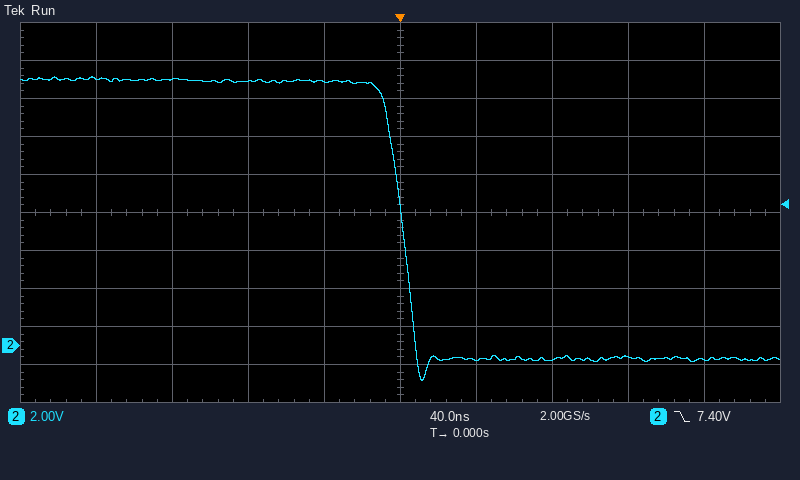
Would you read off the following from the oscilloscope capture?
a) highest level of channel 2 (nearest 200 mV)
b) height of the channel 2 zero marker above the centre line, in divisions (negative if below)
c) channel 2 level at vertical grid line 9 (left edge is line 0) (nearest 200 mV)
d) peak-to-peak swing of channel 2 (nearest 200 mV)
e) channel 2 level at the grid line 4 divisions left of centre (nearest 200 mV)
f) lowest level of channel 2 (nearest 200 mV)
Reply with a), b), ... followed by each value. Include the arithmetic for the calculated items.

a) 14.2 V
b) -3.5 div
c) -800 mV
d) 14.2 V − (-1.8 V) = 16.0 V
e) 14.0 V
f) -1.8 V
